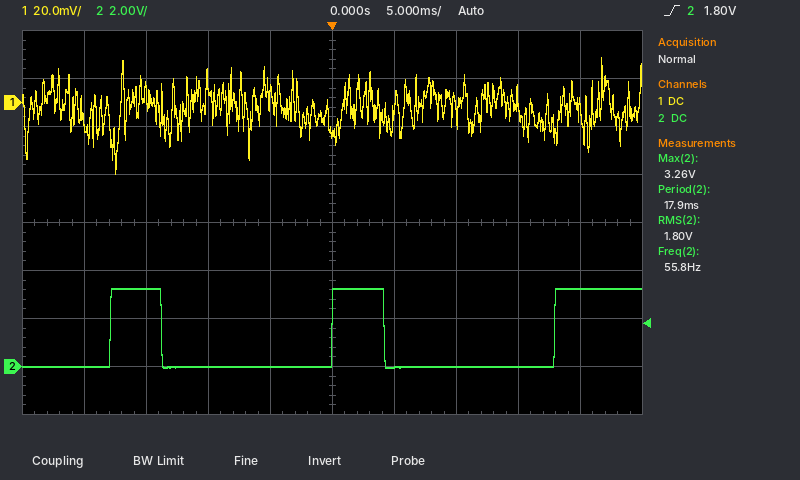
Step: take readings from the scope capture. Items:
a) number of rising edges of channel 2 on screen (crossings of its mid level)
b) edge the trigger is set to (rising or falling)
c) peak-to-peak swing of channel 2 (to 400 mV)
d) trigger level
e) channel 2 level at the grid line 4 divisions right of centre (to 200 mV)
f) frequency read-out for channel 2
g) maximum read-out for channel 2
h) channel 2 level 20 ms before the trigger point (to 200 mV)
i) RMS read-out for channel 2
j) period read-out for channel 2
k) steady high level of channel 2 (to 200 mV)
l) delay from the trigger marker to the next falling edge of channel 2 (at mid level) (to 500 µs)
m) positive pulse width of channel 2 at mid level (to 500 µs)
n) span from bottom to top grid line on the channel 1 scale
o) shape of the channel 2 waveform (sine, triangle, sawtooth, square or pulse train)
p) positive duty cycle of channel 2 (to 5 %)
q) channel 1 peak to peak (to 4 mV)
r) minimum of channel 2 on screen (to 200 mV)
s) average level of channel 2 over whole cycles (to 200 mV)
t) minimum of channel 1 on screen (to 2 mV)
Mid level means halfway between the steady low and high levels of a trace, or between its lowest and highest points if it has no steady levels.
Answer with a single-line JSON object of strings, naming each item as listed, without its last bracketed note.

{"number of rising edges of channel 2 on screen": "3", "edge the trigger is set to": "rising", "peak-to-peak swing of channel 2": "3.2 V", "trigger level": "1.80 V", "channel 2 level at the grid line 4 divisions right of centre": "3.2 V", "frequency read-out for channel 2": "55.8 Hz", "maximum read-out for channel 2": "3.26 V", "channel 2 level 20 ms before the trigger point": "0.0 V", "RMS read-out for channel 2": "1.80 V", "period read-out for channel 2": "17.9 ms", "steady high level of channel 2": "3.2 V", "delay from the trigger marker to the next falling edge of channel 2 (at mid level)": "4.0 ms", "positive pulse width of channel 2 at mid level": "4.0 ms", "span from bottom to top grid line on the channel 1 scale": "160 mV", "shape of the channel 2 waveform": "pulse train", "positive duty cycle of channel 2": "25 %", "channel 1 peak to peak": "48 mV", "minimum of channel 2 on screen": "0.0 V", "average level of channel 2 over whole cycles": "800 mV", "minimum of channel 1 on screen": "-30 mV"}
